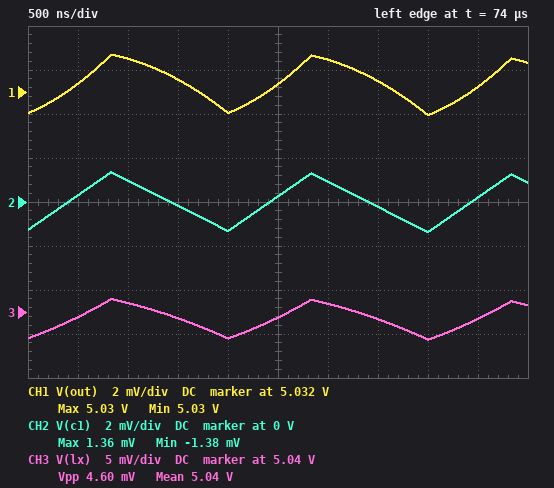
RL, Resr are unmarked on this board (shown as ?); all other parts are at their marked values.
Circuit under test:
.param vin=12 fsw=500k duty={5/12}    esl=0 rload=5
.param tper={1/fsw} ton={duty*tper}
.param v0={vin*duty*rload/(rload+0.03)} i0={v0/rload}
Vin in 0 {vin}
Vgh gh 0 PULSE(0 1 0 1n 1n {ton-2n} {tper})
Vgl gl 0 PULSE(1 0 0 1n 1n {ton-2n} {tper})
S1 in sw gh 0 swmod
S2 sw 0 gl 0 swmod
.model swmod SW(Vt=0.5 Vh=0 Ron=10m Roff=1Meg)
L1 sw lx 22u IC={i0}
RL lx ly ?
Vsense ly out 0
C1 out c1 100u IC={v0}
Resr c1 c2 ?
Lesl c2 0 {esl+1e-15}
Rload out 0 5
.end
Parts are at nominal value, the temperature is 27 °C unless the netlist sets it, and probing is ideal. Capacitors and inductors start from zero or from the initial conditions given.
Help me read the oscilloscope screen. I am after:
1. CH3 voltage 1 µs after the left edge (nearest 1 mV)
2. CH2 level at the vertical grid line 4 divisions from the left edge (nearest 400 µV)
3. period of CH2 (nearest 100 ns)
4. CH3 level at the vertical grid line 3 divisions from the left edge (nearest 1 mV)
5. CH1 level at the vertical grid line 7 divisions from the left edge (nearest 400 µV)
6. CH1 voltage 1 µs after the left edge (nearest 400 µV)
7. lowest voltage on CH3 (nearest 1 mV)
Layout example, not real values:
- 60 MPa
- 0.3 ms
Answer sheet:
- 5.041 V
- -1.2 mV
- 2.0 µs
- 5.039 V
- 5.0324 V
- 5.0336 V
- 5.037 V
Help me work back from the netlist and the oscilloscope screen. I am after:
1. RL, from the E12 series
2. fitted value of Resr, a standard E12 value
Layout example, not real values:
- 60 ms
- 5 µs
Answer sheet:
- 6.8 mΩ
- 0.01 Ω
